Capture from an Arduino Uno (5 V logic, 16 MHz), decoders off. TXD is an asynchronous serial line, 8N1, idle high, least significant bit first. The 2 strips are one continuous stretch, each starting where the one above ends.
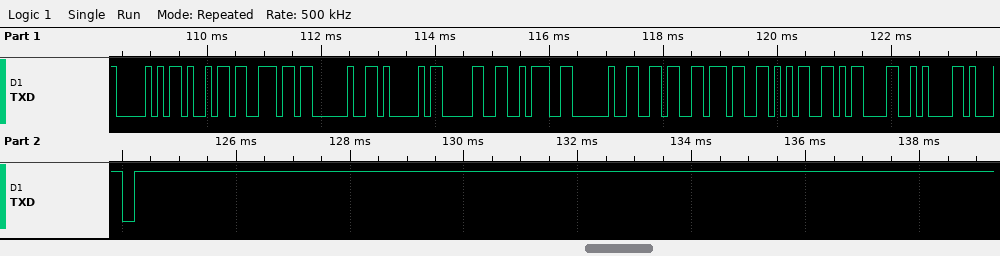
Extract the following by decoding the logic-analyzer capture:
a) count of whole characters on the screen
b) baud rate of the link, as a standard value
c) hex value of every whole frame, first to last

14
9600 baud
0x50 0x69 0x6E 0x20 0x41 0x30 0x3A 0x20 0x36 0x37 0x35 0x0D 0x0A 0x31
